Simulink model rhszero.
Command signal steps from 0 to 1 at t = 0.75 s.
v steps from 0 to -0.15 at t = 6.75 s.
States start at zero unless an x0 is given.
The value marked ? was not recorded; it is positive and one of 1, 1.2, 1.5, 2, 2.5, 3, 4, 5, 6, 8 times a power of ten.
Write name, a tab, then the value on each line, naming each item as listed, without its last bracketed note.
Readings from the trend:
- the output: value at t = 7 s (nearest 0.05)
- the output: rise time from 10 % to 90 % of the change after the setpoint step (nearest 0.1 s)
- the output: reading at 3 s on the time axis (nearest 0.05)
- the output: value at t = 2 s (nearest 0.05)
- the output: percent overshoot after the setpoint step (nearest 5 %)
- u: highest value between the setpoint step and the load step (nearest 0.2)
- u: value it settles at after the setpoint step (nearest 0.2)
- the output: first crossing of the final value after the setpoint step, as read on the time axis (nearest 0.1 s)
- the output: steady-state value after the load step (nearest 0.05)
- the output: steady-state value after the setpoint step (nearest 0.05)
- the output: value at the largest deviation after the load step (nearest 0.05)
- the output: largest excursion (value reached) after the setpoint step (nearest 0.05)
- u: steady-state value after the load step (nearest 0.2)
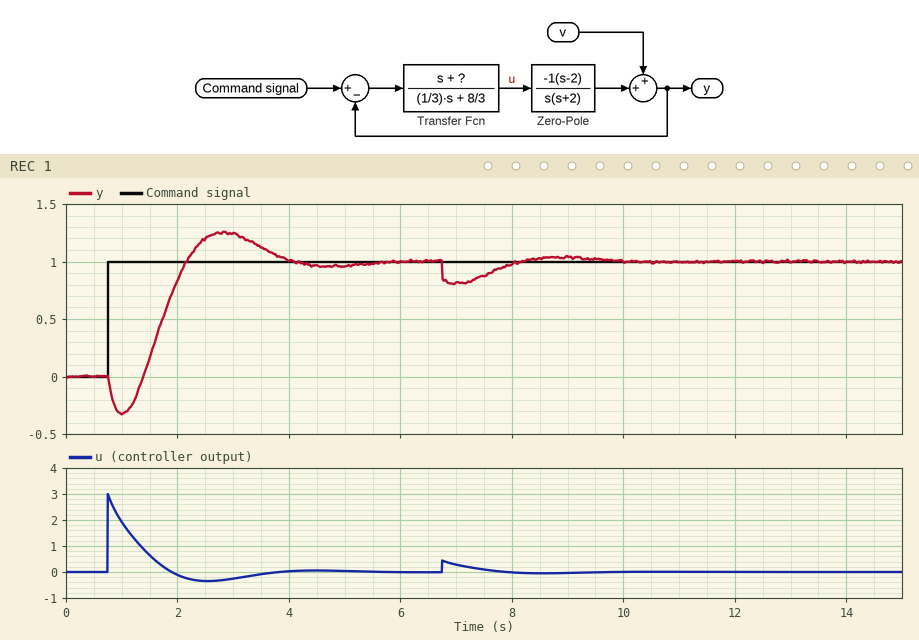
the output: value at t = 7 s	0.80
the output: rise time from 10 % to 90 % of the change after the setpoint step	0.6 s
the output: reading at 3 s on the time axis	1.25
the output: value at t = 2 s	0.85
the output: percent overshoot after the setpoint step	25 %
u: highest value between the setpoint step and the load step	3.0
u: value it settles at after the setpoint step	0.0
the output: first crossing of the final value after the setpoint step, as read on the time axis	2.2 s
the output: steady-state value after the load step	1.00
the output: steady-state value after the setpoint step	1.00
the output: value at the largest deviation after the load step	0.80
the output: largest excursion (value reached) after the setpoint step	1.25
u: steady-state value after the load step	0.0
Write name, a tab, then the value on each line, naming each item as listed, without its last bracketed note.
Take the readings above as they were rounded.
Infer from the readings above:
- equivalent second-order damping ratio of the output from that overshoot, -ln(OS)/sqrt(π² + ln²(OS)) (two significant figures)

equivalent second-order damping ratio of the output from that overshoot, -ln(OS)/sqrt(π² + ln²(OS))	0.40
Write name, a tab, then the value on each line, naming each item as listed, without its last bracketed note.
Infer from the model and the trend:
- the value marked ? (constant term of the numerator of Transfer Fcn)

the value marked ?	3
